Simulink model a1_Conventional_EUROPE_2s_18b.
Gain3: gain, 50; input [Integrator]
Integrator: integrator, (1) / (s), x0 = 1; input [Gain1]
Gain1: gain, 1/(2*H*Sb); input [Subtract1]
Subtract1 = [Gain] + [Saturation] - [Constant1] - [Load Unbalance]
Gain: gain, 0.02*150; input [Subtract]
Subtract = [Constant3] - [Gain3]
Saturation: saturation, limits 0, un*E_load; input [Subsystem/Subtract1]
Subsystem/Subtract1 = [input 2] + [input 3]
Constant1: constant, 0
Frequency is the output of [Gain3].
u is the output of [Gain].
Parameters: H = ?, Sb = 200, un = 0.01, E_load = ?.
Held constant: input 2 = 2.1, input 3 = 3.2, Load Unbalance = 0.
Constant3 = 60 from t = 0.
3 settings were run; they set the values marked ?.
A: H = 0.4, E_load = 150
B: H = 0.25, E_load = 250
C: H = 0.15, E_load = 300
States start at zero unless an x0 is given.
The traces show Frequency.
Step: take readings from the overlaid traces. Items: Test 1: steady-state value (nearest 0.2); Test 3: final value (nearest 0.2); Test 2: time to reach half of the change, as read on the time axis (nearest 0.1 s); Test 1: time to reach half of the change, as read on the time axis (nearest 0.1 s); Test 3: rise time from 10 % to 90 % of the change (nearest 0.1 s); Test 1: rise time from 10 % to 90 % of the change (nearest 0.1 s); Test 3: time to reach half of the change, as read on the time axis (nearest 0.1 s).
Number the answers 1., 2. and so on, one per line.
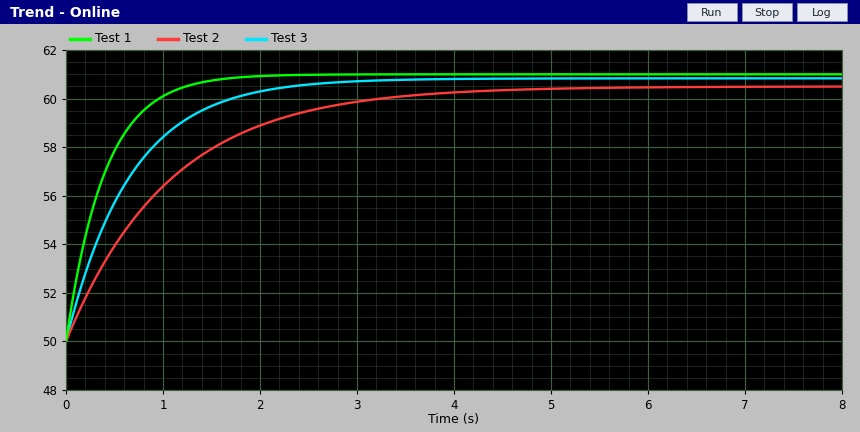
1. 61.0
2. 60.8
3. 0.7 s
4. 0.3 s
5. 1.5 s
6. 0.9 s
7. 0.5 s
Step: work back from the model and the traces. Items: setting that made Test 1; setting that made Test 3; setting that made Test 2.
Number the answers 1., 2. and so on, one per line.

1. C
2. B
3. A
